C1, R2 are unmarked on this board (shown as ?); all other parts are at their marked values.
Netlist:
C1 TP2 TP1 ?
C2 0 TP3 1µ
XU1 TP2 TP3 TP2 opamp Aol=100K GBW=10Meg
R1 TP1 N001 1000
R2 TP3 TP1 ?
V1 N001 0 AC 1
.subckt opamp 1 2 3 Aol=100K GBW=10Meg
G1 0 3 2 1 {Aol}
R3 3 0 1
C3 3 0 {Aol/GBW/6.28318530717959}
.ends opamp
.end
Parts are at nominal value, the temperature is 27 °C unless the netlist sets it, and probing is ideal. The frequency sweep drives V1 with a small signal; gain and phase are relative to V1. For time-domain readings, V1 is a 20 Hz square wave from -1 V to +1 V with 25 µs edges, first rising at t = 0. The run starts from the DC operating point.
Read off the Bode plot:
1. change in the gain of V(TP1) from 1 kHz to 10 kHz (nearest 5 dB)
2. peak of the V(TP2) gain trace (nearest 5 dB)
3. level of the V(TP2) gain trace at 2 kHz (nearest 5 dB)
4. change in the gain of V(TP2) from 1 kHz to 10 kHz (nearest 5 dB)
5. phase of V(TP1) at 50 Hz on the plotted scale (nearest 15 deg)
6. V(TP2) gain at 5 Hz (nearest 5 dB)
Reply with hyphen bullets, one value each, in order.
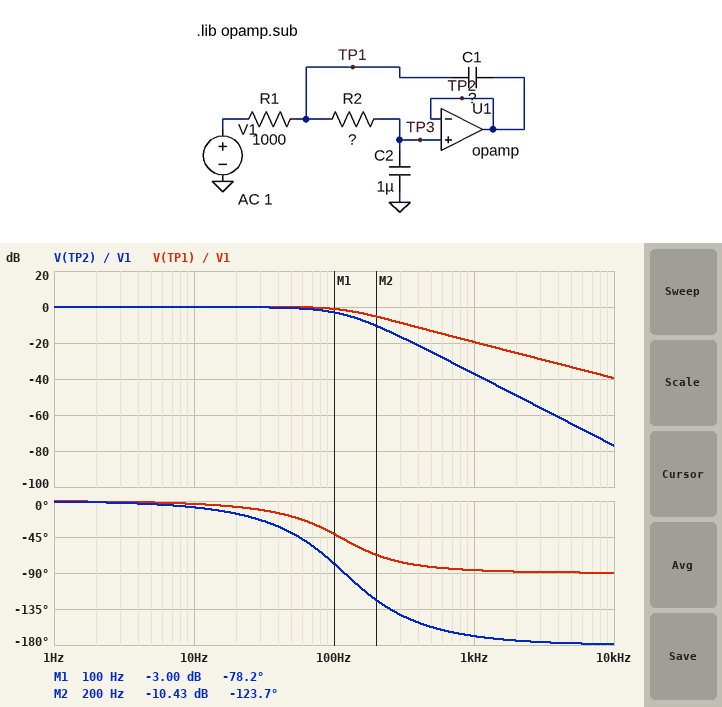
- -20 dB
- 0 dB
- -50 dB
- -40 dB
- -15 deg
- 0 dB
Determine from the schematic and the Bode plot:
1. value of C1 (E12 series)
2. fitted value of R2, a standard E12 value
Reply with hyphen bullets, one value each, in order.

- 1.5 µF
- 1.2 kΩ
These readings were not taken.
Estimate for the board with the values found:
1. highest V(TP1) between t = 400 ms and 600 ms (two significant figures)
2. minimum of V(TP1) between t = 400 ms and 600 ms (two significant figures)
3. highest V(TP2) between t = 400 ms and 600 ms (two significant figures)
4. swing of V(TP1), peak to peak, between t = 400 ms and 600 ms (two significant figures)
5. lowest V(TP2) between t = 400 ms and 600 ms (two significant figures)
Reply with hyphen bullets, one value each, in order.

- 1.1 V
- -1.1 V
- 1.0 V
- 2.1 V
- -1.0 V
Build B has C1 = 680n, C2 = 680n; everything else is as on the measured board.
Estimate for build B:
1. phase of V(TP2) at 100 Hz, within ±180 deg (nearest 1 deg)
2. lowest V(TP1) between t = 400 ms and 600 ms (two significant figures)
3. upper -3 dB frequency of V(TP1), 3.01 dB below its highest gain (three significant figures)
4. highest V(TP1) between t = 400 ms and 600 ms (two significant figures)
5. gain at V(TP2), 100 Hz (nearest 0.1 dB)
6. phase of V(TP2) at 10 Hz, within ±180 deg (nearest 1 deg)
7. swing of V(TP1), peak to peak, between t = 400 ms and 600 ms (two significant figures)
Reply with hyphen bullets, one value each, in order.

- -50 deg
- -1.0 V
- 234 Hz
- 1.0 V
- -1.7 dB
- -5 deg
- 2.0 V
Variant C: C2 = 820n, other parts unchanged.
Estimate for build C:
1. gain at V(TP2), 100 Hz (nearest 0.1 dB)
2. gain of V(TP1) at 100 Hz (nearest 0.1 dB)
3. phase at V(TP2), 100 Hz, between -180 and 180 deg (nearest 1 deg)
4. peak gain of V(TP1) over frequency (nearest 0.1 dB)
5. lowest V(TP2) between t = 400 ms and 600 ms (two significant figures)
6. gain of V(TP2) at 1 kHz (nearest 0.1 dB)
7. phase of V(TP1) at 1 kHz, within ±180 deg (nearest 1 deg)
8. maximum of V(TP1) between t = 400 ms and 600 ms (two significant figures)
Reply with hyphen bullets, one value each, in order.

- -1.6 dB
- -0.2 dB
- -70 deg
- 0.2 dB
- -1.1 V
- -35.3 dB
- -88 deg
- 1.1 V
